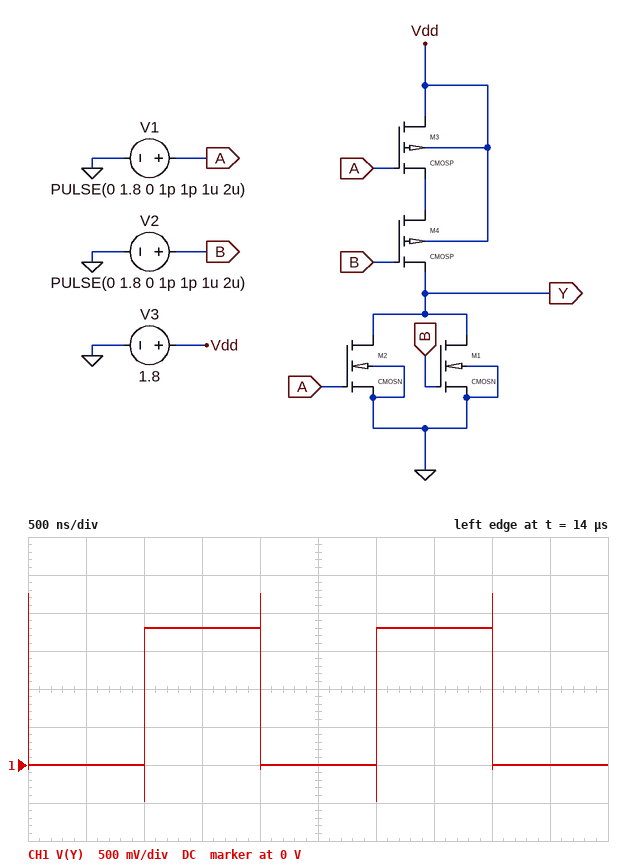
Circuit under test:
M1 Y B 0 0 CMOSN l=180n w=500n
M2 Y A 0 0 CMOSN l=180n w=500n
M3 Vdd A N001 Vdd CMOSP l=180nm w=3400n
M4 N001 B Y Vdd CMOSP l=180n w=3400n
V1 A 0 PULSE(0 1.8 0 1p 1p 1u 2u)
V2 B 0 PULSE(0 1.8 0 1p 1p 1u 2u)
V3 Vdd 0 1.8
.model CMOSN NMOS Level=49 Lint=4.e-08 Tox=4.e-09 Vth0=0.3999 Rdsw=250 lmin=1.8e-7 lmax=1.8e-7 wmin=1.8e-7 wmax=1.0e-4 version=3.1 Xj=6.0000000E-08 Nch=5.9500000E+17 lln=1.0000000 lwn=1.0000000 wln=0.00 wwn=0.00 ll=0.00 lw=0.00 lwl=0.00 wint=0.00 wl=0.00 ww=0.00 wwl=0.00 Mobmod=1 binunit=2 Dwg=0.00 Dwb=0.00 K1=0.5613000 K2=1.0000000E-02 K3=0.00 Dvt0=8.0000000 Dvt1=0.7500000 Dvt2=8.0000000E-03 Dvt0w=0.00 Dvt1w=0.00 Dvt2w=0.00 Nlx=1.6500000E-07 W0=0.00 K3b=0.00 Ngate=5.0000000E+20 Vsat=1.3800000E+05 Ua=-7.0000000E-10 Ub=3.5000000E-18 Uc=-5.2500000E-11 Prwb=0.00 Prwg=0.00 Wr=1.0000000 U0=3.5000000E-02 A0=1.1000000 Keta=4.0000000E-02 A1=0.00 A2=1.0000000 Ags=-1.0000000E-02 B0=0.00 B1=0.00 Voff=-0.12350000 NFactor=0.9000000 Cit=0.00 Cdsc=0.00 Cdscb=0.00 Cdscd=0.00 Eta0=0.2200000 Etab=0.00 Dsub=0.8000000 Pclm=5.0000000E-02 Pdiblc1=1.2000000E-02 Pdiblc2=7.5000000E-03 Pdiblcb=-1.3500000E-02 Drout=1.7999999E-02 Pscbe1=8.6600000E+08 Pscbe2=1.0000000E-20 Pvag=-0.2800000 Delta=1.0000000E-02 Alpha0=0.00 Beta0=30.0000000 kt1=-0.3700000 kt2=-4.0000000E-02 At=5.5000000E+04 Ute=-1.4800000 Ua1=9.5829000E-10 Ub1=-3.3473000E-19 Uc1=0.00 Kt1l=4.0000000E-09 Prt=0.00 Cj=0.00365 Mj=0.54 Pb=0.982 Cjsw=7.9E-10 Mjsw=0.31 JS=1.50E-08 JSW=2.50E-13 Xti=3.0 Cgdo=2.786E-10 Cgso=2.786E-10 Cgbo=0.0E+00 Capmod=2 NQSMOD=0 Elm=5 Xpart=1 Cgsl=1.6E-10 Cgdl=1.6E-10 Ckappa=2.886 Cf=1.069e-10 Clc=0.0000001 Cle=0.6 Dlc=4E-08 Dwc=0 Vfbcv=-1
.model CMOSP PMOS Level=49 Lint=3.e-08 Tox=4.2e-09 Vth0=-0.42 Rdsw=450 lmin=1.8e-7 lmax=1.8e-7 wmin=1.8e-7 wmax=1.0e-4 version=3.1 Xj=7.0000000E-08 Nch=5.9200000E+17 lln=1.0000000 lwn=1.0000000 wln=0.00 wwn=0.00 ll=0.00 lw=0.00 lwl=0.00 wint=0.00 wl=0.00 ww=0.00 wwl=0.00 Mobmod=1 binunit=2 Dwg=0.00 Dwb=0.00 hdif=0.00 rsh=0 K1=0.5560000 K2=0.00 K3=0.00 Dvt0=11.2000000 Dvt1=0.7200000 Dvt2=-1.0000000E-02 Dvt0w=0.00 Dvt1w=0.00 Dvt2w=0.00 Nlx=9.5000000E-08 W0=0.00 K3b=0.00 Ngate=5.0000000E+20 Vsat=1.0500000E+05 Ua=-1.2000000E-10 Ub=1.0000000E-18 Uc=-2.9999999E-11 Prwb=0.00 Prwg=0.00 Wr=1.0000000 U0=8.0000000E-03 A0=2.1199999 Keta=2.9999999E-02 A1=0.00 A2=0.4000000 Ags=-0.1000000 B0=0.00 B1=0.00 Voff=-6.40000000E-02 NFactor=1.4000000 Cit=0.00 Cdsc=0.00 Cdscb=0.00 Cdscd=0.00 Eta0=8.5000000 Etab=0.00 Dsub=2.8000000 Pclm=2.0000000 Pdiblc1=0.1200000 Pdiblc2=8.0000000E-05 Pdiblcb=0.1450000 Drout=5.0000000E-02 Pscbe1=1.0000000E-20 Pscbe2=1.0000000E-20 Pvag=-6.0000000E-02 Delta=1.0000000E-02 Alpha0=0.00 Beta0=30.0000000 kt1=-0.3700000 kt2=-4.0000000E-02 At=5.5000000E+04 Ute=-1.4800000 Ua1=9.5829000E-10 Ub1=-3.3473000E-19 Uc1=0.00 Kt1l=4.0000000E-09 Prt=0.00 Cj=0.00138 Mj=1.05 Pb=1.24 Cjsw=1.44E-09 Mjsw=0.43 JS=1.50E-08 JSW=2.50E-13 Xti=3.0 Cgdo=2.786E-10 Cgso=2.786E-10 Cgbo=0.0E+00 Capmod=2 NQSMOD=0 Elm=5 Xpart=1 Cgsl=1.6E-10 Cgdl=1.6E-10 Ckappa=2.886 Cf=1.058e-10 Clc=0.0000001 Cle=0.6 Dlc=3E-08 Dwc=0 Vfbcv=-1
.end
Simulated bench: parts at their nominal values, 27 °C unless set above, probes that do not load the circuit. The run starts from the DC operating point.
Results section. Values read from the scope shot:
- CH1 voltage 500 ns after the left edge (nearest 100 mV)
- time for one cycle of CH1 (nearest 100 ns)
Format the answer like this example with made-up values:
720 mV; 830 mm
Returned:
0 V; 2.0 µs
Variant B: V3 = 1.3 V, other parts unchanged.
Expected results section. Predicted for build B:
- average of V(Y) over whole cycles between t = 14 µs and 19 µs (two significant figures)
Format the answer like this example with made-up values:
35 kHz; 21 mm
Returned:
650 mV
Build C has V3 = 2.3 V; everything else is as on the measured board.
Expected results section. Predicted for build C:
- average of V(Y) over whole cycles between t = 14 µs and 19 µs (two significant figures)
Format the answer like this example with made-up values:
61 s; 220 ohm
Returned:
1.2 V
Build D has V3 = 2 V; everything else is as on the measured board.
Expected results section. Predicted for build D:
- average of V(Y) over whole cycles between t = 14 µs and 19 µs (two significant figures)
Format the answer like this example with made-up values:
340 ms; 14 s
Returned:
1.0 V
